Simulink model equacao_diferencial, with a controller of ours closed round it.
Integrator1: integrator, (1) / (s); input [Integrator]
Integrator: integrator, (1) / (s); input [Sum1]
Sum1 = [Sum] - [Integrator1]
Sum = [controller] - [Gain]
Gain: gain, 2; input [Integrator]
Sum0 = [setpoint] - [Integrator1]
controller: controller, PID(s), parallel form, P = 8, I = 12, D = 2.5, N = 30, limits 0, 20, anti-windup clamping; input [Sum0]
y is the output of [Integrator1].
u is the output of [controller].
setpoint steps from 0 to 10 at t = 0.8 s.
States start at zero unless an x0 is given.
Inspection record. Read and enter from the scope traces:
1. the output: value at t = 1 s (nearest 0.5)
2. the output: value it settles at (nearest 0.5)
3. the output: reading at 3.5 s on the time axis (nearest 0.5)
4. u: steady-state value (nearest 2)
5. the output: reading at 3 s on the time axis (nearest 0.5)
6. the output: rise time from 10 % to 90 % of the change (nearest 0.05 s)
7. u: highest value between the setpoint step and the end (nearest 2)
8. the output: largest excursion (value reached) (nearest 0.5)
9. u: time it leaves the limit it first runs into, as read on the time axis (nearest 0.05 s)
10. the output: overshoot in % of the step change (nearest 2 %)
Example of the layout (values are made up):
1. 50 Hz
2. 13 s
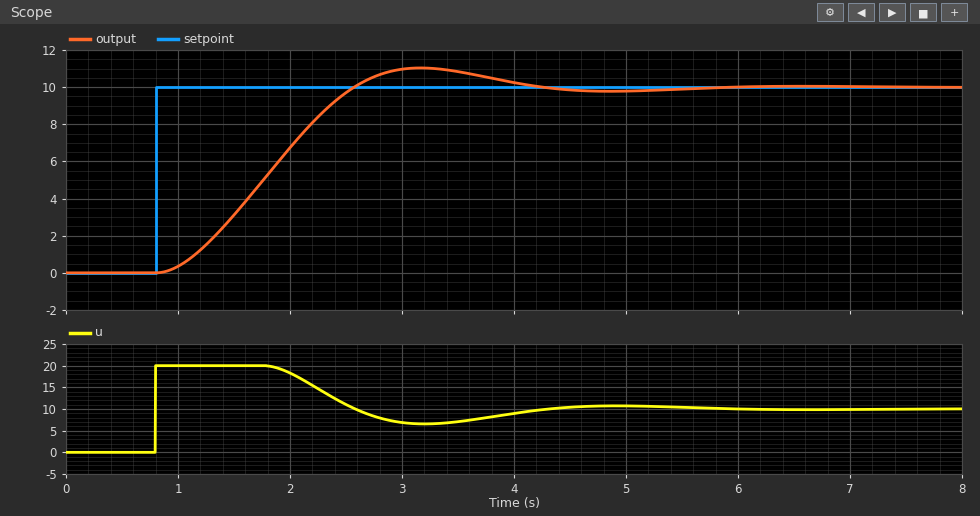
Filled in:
1. 0.5
2. 10.0
3. 11.0
4. 10
5. 11.0
6. 1.20 s
7. 20
8. 11.0
9. 1.85 s
10. 10 %
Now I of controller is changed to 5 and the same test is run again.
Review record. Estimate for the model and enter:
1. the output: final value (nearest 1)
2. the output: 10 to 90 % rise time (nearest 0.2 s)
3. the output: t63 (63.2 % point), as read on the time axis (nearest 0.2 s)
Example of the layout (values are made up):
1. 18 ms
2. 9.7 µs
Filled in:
1. 10
2. 1.4 s
3. 2.0 s
